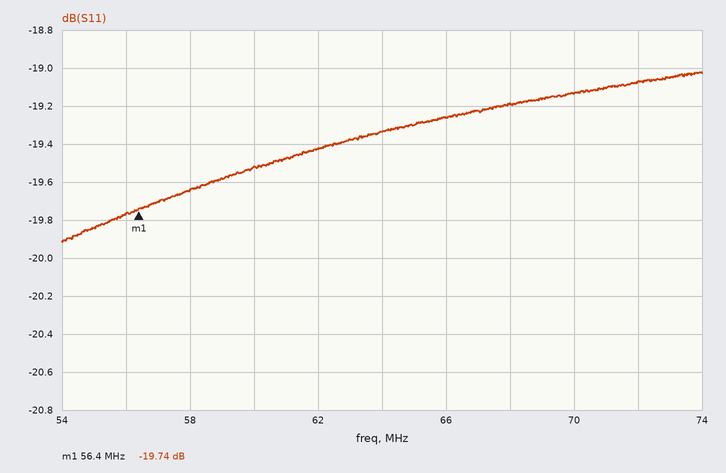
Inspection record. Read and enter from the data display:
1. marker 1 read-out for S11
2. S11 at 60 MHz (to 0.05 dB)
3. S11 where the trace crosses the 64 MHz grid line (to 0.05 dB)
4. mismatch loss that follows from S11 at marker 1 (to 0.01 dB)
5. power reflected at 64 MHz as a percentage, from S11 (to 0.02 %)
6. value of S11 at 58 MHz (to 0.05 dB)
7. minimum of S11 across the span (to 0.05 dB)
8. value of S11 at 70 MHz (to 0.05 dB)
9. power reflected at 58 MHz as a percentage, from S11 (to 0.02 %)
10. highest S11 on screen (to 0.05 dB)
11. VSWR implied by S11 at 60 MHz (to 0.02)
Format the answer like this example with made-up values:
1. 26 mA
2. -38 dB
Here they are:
1. -19.74 dB
2. -19.50 dB
3. -19.35 dB
4. 0.05 dB
5. 1.16 %
6. -19.65 dB
7. -19.90 dB
8. -19.15 dB
9. 1.08 %
10. -19.00 dB
11. 1.24
